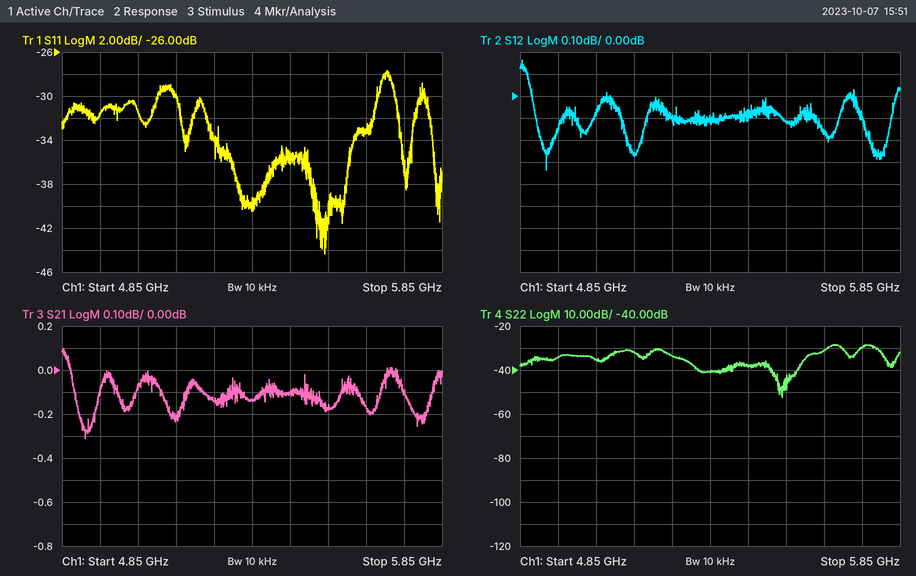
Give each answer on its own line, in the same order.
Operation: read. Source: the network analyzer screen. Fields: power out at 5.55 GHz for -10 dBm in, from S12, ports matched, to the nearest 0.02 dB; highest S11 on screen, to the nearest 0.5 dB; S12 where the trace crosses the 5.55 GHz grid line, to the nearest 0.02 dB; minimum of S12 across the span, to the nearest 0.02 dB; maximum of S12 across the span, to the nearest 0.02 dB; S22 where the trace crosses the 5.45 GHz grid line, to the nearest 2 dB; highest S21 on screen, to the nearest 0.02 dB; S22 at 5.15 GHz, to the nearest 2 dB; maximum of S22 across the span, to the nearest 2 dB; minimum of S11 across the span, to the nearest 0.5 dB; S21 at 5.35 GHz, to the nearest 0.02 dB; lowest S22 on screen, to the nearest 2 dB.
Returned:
-10.12 dBm
-27.5 dB
-0.12 dB
-0.34 dB
0.16 dB
-38 dB
0.10 dB
-32 dB
-28 dB
-44.5 dB
-0.14 dB
-52 dB
